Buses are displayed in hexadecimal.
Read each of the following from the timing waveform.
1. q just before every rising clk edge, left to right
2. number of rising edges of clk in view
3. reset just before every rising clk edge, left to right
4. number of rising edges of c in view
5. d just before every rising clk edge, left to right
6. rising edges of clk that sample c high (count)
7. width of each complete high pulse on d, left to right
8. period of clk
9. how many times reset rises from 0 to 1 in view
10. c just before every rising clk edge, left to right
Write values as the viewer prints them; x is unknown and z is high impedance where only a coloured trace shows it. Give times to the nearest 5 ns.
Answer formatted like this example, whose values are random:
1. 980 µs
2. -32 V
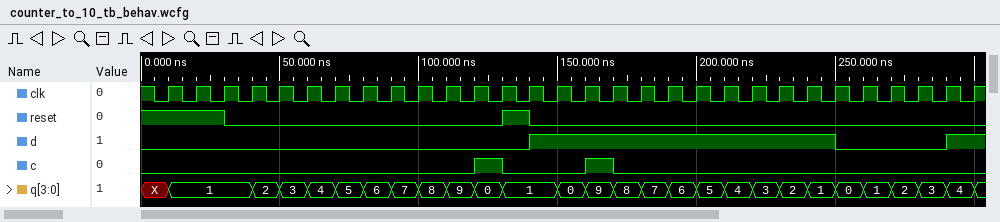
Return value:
1. X, 1, 1, 1, 2, 3, 4, 5, 6, 7, 8, 9, 0, 1, 1, 0, 9, 8, 7, 6, 5, 4, 3, 2, 1, 0, 1, 2, 3, 4
2. 30
3. 1 1 1 0 0 0 0 0 0 0 0 0 0 1 0 0 0 0 0 0 0 0 0 0 0 0 0 0 0 0
4. 2
5. 0 0 0 0 0 0 0 0 0 0 0 0 0 0 1 1 1 1 1 1 1 1 1 1 1 0 0 0 0 1
6. 2
7. 110 ns
8. 10 ns
9. 1
10. 0 0 0 0 0 0 0 0 0 0 0 0 1 0 0 0 1 0 0 0 0 0 0 0 0 0 0 0 0 0
